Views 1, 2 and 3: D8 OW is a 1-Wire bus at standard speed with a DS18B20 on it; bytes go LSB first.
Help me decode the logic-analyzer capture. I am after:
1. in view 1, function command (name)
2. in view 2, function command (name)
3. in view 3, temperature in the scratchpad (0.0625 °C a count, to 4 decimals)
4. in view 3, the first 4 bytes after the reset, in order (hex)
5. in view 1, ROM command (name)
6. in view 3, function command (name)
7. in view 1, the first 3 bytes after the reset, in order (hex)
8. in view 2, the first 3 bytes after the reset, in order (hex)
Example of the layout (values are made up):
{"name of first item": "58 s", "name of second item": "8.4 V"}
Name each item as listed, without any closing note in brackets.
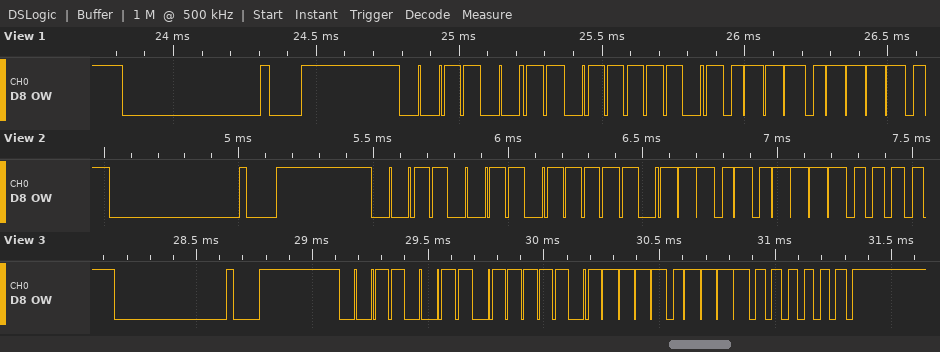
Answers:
{"in view 1, function command": "Read Scratchpad", "in view 2, function command": "Read Scratchpad", "in view 3, temperature in the scratchpad": "30.9375 °C", "in view 3, the first 4 bytes after the reset, in order": "CC BE EF 01", "in view 1, ROM command": "Skip ROM", "in view 3, function command": "Read Scratchpad", "in view 1, the first 3 bytes after the reset, in order": "CC BE EE", "in view 2, the first 3 bytes after the reset, in order": "CC BE EB"}
